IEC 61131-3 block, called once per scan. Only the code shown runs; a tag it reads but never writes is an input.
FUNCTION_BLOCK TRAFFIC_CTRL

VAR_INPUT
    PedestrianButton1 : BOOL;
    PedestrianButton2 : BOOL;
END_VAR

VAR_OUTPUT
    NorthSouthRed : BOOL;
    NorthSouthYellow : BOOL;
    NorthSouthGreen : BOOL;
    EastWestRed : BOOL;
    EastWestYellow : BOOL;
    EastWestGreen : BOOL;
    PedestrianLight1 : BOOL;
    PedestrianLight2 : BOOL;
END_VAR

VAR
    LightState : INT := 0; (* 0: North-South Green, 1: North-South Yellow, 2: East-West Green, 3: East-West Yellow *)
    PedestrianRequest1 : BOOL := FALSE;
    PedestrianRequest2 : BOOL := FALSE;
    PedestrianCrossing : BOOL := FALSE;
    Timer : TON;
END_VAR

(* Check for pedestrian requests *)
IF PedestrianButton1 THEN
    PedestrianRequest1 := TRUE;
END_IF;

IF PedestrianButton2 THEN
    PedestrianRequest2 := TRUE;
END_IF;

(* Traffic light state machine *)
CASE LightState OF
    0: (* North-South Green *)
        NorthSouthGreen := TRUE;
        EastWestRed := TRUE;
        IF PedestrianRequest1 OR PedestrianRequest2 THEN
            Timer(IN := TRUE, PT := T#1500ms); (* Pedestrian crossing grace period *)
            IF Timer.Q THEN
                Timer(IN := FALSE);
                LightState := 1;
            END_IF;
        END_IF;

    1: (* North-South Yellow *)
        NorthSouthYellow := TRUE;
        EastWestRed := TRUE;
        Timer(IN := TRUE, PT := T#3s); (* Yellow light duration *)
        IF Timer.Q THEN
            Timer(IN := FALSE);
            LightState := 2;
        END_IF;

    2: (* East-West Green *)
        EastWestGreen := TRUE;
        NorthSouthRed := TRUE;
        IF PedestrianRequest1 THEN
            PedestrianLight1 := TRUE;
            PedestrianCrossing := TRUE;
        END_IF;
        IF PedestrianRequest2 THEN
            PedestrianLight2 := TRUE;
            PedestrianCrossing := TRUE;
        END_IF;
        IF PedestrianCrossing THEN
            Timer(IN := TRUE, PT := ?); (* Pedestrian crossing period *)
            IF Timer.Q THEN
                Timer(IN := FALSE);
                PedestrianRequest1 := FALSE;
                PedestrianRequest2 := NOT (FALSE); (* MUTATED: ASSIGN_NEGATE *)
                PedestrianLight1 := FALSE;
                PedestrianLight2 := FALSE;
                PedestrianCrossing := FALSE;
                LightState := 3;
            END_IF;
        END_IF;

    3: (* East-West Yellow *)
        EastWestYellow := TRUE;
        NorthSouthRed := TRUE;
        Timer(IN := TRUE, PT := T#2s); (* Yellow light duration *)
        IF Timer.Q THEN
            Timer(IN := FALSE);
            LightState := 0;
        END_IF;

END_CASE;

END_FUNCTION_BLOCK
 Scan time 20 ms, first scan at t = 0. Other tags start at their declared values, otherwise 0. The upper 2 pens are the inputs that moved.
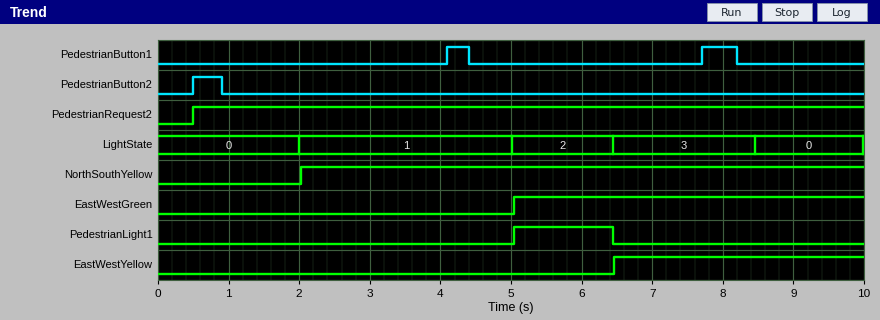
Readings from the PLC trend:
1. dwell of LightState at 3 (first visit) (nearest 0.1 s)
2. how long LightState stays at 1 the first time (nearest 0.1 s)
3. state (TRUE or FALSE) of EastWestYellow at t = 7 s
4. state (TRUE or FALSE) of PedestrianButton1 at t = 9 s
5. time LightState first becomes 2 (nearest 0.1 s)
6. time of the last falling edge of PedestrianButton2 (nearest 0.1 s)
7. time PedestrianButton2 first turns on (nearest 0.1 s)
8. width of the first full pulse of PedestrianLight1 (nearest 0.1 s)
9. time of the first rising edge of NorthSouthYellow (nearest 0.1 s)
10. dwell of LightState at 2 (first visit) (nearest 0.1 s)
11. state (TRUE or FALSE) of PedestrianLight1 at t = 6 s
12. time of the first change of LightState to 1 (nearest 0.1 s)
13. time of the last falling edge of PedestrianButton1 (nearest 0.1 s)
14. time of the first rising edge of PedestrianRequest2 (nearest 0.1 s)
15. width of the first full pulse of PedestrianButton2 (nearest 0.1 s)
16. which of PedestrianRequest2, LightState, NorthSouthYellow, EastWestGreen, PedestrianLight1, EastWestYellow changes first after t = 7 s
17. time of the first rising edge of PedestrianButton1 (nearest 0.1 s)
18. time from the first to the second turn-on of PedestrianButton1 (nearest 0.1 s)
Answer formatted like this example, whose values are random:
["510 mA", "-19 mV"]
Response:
["2.0 s", "3.0 s", "TRUE", "FALSE", "5.0 s", "0.9 s", "0.5 s", "1.4 s", "2.0 s", "1.4 s", "TRUE", "2.0 s", "8.2 s", "0.5 s", "0.4 s", "LightState", "4.1 s", "3.6 s"]
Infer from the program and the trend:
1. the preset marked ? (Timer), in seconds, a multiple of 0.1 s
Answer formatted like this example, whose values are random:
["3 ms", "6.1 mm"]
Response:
["1.4 s"]
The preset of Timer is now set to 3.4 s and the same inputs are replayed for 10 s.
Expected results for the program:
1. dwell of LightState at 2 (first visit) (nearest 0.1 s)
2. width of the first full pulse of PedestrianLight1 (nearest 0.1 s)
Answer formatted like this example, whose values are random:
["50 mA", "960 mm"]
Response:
["3.4 s", "3.4 s"]
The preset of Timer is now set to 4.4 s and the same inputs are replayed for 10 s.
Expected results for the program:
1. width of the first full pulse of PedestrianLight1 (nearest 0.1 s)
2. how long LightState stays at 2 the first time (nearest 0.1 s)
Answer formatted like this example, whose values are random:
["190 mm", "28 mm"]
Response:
["4.4 s", "4.4 s"]
